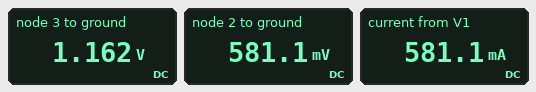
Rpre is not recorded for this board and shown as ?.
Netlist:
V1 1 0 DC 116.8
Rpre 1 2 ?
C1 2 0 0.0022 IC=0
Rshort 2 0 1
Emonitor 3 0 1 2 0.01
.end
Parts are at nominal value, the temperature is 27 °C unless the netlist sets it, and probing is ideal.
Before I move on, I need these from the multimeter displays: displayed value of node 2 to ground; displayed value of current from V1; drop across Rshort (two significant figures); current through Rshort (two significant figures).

581.1 mV
581.1 mA
580 mV
580 mA
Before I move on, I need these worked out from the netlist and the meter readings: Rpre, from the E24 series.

200 Ω
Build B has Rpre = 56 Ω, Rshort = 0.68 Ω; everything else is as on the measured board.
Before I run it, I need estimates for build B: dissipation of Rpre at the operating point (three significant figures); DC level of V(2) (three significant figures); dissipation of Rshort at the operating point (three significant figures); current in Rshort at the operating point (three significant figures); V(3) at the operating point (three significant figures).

238 W
1.40 V
2.89 W
2.06 A
1.15 V
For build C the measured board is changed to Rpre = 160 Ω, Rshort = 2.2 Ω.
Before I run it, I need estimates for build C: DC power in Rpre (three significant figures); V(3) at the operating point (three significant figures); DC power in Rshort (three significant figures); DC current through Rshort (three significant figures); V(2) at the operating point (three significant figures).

83.0 W
1.15 V
1.14 W
720 mA
1.58 V
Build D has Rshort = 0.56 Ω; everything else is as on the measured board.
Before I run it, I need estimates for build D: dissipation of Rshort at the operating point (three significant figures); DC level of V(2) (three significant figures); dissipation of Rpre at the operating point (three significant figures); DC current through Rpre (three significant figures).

190 mW
326 mV
67.8 W
582 mA
